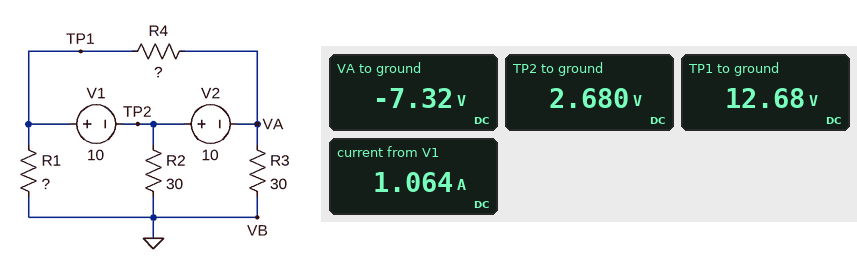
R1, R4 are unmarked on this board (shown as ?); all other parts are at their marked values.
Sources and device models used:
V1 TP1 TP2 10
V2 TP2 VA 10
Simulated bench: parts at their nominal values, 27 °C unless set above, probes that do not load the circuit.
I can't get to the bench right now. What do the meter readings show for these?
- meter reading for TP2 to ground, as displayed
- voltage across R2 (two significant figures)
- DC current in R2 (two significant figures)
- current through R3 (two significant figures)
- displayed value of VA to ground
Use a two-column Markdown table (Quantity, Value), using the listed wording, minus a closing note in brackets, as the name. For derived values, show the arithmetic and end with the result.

| Quantity | Value |
|---|---|
| meter reading for TP2 to ground, as displayed | 2.680 V |
| voltage across R2 | 2.68 V = 2.7 V |
| DC current in R2 | (2.68 V) / 30 Ω = 89 mA |
| current through R3 | (0 V - (-7.32 V)) / 30 Ω = 240 mA |
| displayed value of VA to ground | -7.32 V |
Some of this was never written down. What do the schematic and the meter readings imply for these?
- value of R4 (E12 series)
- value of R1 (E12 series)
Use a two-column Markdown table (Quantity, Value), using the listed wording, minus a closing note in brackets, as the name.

| Quantity | Value |
|---|---|
| value of R4 | 22 Ω |
| value of R1 | 82 Ω |
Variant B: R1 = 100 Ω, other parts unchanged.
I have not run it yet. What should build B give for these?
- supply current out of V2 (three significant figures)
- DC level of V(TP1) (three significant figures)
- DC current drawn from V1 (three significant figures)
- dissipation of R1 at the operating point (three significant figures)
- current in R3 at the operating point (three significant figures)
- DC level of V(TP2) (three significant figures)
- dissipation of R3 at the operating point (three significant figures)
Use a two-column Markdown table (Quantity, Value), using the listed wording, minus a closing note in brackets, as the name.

| Quantity | Value |
|---|---|
| supply current out of V2 | 1.14 A |
| DC level of V(TP1) | 13.0 V |
| DC current drawn from V1 | 1.04 A |
| dissipation of R1 at the operating point | 1.70 W |
| current in R3 at the operating point | 232 mA |
| DC level of V(TP2) | 3.04 V |
| dissipation of R3 at the operating point | 1.61 W |
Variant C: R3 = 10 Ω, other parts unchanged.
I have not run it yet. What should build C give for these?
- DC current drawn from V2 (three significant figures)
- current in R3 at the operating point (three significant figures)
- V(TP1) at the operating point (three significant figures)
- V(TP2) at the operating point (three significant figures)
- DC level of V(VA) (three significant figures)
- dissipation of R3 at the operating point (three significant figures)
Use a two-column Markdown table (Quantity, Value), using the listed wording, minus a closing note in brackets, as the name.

| Quantity | Value |
|---|---|
| DC current drawn from V2 | 1.31 A |
| current in R3 at the operating point | 397 mA |
| V(TP1) at the operating point | 16.0 V |
| V(TP2) at the operating point | 6.03 V |
| DC level of V(VA) | -3.97 V |
| dissipation of R3 at the operating point | 1.57 W |
